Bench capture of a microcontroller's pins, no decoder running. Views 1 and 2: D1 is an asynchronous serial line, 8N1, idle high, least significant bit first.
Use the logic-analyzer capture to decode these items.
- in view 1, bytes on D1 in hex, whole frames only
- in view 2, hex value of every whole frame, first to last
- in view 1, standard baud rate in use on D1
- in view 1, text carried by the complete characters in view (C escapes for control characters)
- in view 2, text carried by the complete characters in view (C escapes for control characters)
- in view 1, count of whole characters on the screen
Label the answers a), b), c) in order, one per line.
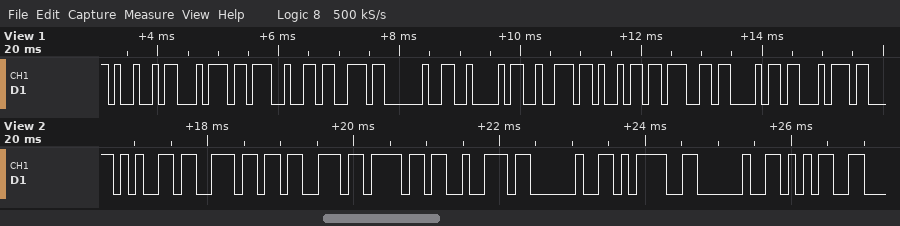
a) 0x49 0x74 0x27 0x73 0x20 0x42 0x72 0x69 0x67 0x68 0x74
b) 0x65 0x6E 0x73 0x6F 0x72 0x20 0x3D 0x20 0x35
c) 9600 baud
d) "It's Bright"
e) "ensor = 5"
f) 11
